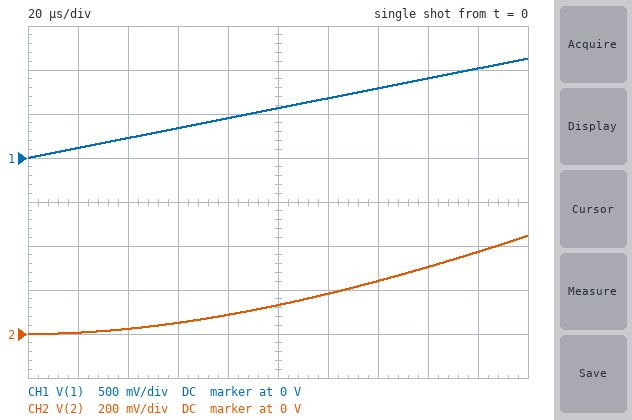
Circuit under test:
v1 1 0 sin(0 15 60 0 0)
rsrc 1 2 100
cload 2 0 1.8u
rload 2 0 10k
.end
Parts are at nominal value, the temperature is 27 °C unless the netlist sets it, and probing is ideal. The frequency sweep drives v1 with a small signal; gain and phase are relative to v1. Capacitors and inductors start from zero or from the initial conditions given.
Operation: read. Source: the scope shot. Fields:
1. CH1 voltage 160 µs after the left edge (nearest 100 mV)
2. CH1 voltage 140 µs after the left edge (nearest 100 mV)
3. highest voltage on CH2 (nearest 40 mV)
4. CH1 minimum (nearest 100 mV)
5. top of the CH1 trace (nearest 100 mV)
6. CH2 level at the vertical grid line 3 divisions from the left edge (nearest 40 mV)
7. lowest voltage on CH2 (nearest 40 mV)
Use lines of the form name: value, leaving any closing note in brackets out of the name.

CH1 voltage 160 µs after the left edge: 900 mV
CH1 voltage 140 µs after the left edge: 800 mV
highest voltage on CH2: 440 mV
CH1 minimum: 0 V
top of the CH1 trace: 1.1 V
CH2 level at the vertical grid line 3 divisions from the left edge: 40 mV
lowest voltage on CH2: 0 V
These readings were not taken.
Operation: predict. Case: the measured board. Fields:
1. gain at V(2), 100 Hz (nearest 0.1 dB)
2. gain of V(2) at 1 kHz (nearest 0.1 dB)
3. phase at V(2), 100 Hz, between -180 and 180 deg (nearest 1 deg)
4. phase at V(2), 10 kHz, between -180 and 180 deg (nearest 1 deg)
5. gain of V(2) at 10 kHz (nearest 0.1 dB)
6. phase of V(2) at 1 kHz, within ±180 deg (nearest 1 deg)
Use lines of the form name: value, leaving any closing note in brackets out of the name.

gain at V(2), 100 Hz: -0.1 dB
gain of V(2) at 1 kHz: -3.6 dB
phase at V(2), 100 Hz, between -180 and 180 deg: -6 deg
phase at V(2), 10 kHz, between -180 and 180 deg: -85 deg
gain of V(2) at 10 kHz: -21.1 dB
phase of V(2) at 1 kHz, within ±180 deg: -48 deg
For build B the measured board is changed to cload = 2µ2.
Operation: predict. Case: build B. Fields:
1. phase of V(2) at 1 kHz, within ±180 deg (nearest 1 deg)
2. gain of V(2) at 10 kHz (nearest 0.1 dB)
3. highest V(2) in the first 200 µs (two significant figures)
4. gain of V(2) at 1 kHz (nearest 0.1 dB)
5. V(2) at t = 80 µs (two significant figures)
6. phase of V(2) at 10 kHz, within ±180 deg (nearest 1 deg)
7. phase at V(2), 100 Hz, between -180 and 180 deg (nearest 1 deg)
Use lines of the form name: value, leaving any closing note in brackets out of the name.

phase of V(2) at 1 kHz, within ±180 deg: -54 deg
gain of V(2) at 10 kHz: -22.8 dB
highest V(2) in the first 200 µs: 390 mV
gain of V(2) at 1 kHz: -4.7 dB
V(2) at t = 80 µs: 73 mV
phase of V(2) at 10 kHz, within ±180 deg: -86 deg
phase at V(2), 100 Hz, between -180 and 180 deg: -8 deg
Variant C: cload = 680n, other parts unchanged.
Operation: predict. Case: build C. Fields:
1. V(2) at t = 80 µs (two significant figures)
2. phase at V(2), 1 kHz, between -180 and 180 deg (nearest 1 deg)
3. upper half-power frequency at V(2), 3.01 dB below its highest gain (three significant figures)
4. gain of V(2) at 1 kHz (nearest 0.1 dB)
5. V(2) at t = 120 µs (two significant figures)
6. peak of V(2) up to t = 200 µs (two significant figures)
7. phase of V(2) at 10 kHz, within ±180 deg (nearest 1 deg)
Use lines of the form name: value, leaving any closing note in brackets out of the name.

V(2) at t = 80 µs: 190 mV
phase at V(2), 1 kHz, between -180 and 180 deg: -23 deg
upper half-power frequency at V(2), 3.01 dB below its highest gain: 2.36 kHz
gain of V(2) at 1 kHz: -0.8 dB
V(2) at t = 120 µs: 360 mV
peak of V(2) up to t = 200 µs: 760 mV
phase of V(2) at 10 kHz, within ±180 deg: -77 deg
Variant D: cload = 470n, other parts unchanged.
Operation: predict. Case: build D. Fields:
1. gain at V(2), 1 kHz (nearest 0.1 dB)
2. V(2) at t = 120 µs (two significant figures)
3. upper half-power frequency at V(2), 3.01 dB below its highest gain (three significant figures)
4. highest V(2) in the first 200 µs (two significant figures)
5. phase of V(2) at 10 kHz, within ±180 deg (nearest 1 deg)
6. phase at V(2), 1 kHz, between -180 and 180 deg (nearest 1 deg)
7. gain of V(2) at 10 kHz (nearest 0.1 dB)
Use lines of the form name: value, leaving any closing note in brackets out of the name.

gain at V(2), 1 kHz: -0.4 dB
V(2) at t = 120 µs: 430 mV
upper half-power frequency at V(2), 3.01 dB below its highest gain: 3.42 kHz
highest V(2) in the first 200 µs: 860 mV
phase of V(2) at 10 kHz, within ±180 deg: -71 deg
phase at V(2), 1 kHz, between -180 and 180 deg: -16 deg
gain of V(2) at 10 kHz: -9.9 dB
